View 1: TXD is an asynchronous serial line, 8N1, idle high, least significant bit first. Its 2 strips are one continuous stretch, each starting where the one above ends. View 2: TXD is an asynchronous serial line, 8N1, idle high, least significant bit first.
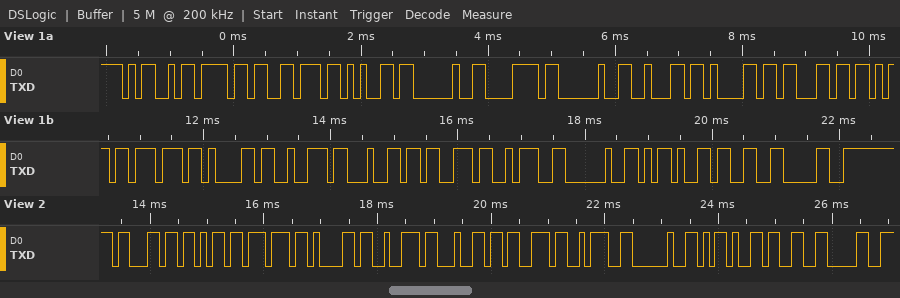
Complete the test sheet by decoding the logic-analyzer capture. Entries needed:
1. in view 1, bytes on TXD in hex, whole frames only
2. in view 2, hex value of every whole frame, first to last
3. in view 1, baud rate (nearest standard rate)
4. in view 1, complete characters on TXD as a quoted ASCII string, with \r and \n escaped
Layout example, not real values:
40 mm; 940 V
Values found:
4D 6F 76 65 20 78 20 62 61 63 6B 77 61 72 64 73 3A 20 2D 33 30; 63 6B 77 61 72 64 73 3A 20 2D 33 30; 9600 baud; "Move x backwards: -30"
